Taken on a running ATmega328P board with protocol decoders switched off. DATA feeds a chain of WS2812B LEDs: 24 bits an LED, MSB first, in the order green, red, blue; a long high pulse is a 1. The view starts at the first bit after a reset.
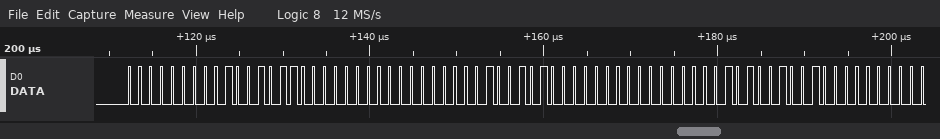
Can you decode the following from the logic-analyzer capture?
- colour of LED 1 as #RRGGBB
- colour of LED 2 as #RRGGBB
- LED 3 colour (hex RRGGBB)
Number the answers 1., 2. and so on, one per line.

1. #4B0000
2. #4A0000
3. #490100
